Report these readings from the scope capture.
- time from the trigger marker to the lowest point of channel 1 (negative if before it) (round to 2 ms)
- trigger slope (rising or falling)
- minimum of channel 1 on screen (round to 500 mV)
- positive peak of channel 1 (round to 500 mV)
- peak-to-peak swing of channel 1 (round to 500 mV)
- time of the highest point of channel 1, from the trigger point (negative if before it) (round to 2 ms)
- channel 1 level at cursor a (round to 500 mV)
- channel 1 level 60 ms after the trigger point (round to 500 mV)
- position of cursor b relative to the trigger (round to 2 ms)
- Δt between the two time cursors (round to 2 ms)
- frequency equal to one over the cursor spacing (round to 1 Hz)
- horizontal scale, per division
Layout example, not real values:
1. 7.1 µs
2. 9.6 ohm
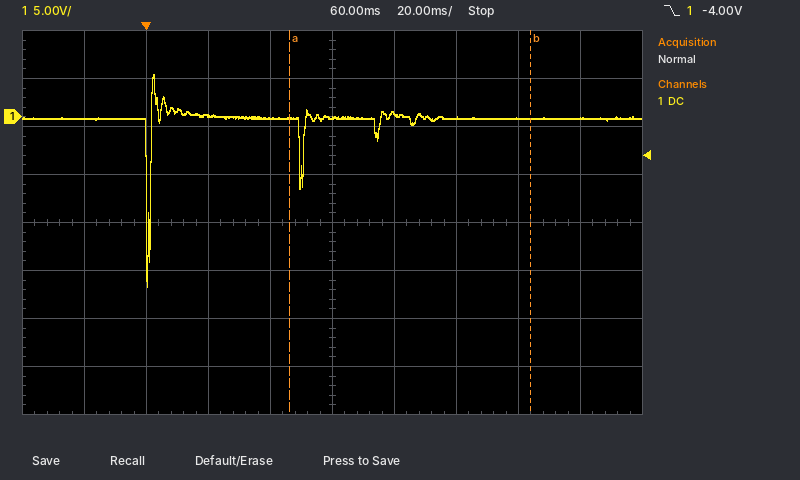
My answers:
1. 0 ms
2. falling
3. -17.5 V
4. 4.5 V
5. 22.0 V
6. +2 ms
7. 0.0 V
8. 0.0 V
9. +124 ms
10. 78 ms
11. 13 Hz
12. 20 ms
